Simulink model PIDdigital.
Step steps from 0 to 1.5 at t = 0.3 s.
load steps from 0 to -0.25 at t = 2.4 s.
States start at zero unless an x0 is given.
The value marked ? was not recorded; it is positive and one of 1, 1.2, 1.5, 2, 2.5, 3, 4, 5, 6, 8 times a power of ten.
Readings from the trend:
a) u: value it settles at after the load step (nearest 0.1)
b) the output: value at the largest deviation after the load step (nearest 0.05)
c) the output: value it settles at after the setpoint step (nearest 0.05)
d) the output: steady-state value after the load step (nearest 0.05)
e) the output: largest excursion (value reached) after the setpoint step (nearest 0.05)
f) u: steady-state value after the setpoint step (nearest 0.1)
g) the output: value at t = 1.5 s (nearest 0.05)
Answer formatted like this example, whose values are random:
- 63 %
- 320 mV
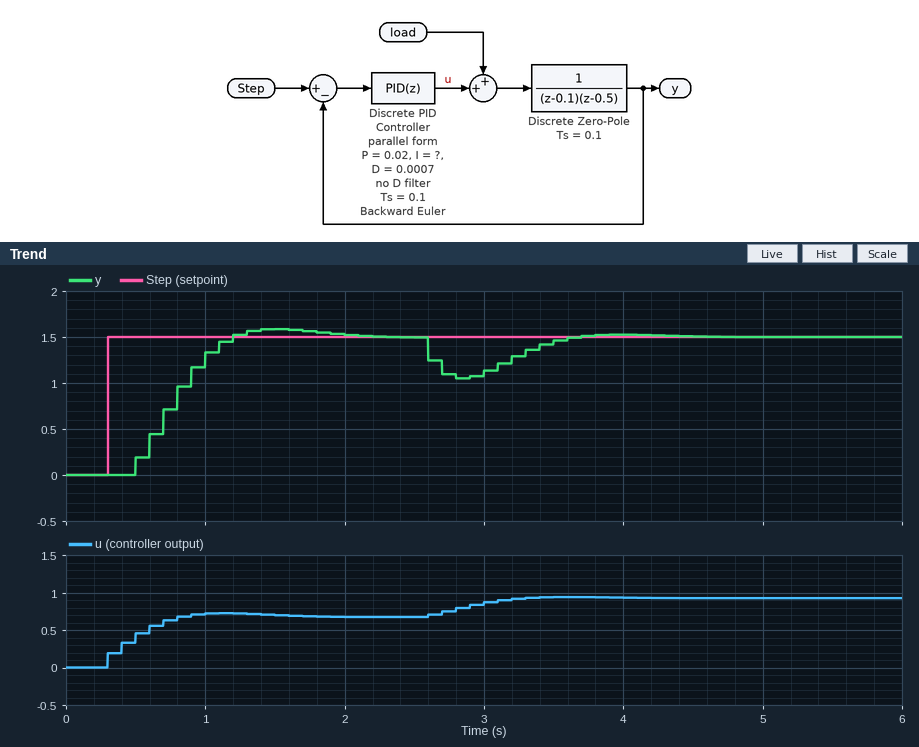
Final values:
- 0.9
- 1.05
- 1.50
- 1.50
- 1.60
- 0.7
- 1.60
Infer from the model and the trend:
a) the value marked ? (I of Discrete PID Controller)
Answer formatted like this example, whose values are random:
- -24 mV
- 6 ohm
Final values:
- 1
